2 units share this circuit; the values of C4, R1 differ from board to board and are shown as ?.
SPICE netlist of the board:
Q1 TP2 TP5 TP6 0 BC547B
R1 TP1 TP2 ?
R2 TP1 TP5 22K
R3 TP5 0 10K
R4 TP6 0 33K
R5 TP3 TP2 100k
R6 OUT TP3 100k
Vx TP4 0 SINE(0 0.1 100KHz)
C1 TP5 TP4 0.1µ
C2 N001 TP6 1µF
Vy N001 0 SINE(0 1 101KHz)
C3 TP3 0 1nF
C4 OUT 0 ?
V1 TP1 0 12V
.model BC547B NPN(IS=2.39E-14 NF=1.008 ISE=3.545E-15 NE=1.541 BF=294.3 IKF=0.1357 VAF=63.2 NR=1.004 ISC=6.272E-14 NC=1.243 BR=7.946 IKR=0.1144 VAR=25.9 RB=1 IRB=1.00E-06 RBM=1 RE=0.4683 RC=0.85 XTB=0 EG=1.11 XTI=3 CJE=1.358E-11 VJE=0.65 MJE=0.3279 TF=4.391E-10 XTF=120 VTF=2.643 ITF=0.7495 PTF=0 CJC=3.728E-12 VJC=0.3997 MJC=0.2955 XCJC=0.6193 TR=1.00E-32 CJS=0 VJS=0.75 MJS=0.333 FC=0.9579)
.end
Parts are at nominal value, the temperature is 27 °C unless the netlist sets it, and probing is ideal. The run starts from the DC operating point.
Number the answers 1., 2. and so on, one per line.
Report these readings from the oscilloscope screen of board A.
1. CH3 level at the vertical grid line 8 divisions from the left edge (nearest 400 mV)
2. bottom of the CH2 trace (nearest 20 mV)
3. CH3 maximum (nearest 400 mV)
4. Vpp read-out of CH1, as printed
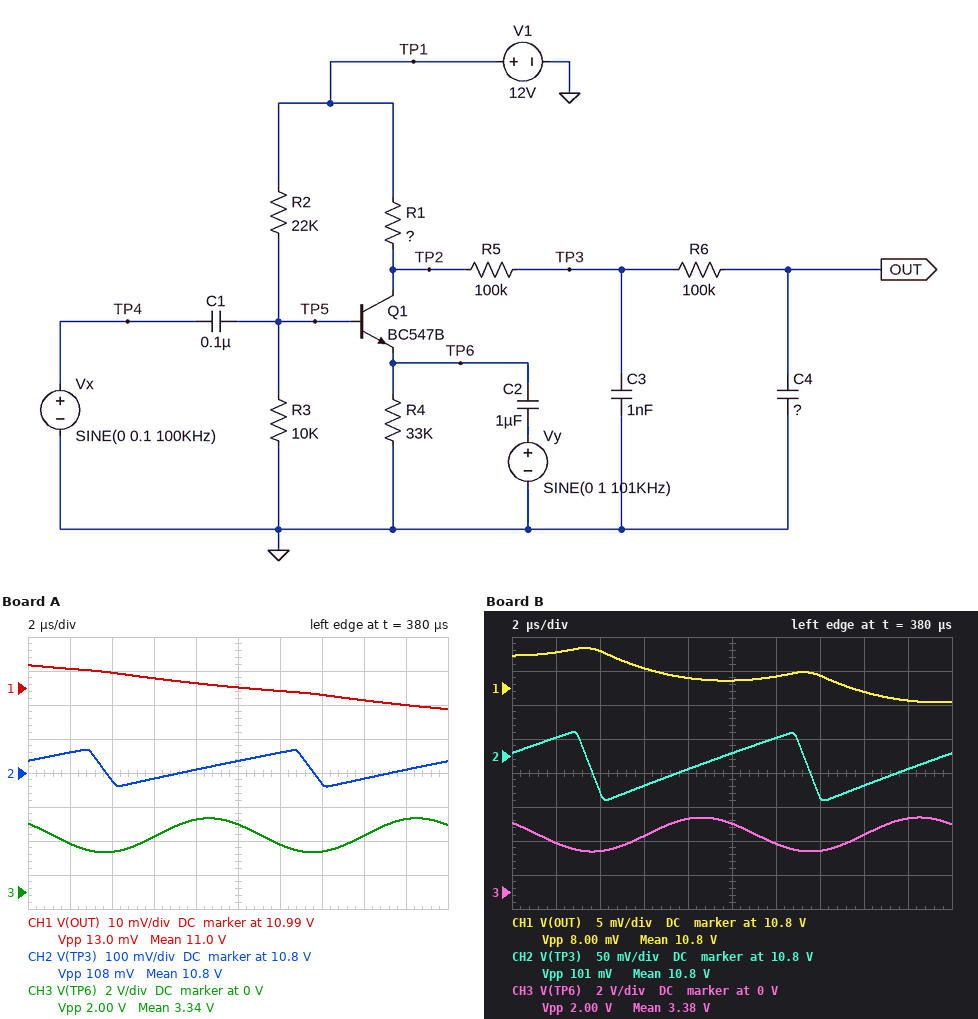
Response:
1. 3.2 V
2. 10.76 V
3. 4.4 V
4. 13.0 mV
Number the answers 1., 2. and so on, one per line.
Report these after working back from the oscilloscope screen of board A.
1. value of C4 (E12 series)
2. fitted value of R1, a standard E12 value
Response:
1. 2.7 nF
2. 6.8 kΩ
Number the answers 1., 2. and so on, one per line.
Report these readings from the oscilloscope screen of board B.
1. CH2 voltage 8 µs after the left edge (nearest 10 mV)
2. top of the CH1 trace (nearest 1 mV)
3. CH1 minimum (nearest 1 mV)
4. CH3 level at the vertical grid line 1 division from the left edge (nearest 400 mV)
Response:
1. 10.78 V
2. 10.806 V
3. 10.798 V
4. 2.8 V
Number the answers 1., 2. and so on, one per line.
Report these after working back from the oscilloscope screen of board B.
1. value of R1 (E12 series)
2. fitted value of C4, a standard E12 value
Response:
1. 3.9 kΩ
2. 470 pF
